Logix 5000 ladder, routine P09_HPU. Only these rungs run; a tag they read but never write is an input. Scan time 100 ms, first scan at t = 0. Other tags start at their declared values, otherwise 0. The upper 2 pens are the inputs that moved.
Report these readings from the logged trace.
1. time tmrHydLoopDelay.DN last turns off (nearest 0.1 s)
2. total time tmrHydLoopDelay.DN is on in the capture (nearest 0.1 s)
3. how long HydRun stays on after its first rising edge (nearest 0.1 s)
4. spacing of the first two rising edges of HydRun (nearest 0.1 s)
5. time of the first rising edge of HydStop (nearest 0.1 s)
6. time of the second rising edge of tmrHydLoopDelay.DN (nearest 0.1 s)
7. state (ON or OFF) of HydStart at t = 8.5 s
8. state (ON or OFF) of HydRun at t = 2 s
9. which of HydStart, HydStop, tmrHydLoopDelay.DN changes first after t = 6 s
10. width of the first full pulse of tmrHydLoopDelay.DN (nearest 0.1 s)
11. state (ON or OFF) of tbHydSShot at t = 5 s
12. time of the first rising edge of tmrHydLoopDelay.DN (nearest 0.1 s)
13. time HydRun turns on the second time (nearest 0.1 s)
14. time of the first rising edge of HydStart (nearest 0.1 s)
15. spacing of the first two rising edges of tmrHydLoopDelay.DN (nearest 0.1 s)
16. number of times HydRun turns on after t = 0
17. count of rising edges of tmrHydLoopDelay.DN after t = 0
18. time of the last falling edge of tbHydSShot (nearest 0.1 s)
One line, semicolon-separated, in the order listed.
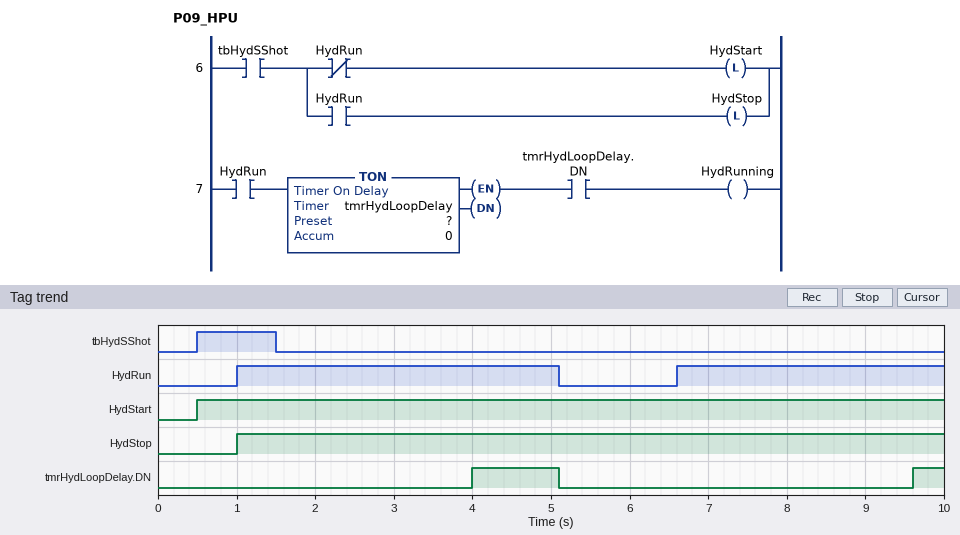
5.1 s; 1.5 s; 4.1 s; 5.6 s; 1.0 s; 9.6 s; ON; ON; tmrHydLoopDelay.DN; 1.1 s; OFF; 4.0 s; 6.6 s; 0.5 s; 5.6 s; 2; 2; 1.5 s
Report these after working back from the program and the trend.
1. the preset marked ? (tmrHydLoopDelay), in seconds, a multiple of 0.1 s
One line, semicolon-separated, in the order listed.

3.0 s
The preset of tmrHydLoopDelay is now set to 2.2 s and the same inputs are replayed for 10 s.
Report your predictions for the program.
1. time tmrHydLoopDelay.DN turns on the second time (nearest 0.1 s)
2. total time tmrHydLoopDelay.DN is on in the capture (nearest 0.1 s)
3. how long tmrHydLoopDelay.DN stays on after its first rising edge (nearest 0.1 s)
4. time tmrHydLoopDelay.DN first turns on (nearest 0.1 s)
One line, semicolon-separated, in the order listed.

8.8 s; 3.1 s; 1.9 s; 3.2 s
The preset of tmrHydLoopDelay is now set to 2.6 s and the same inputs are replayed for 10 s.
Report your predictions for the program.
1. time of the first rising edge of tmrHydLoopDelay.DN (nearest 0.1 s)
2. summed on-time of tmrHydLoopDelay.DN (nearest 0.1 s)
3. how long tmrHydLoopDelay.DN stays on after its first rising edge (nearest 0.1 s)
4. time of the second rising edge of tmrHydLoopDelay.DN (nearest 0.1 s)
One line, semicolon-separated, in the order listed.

3.6 s; 2.3 s; 1.5 s; 9.2 s
